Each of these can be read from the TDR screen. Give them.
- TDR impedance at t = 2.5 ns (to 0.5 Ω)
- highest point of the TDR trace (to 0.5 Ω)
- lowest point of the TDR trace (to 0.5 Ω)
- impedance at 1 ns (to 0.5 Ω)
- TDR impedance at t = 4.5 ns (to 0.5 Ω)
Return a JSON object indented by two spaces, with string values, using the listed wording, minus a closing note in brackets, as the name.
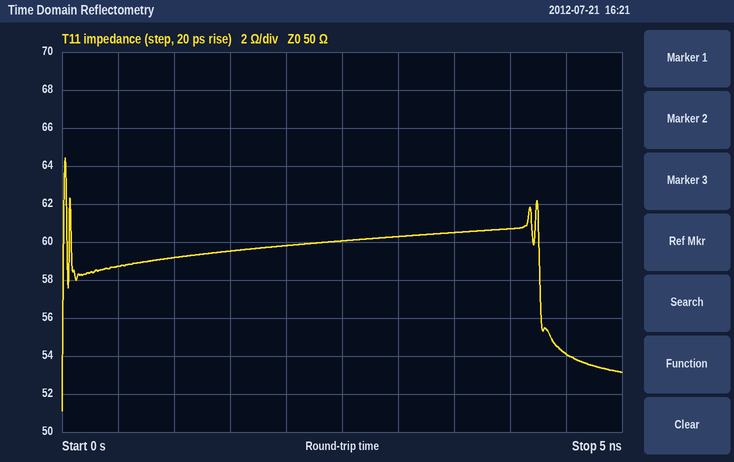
{
  "TDR impedance at t = 2.5 ns": "60.0 Ω",
  "highest point of the TDR trace": "64.5 Ω",
  "lowest point of the TDR trace": "51.0 Ω",
  "impedance at 1 ns": "59.0 Ω",
  "TDR impedance at t = 4.5 ns": "54.0 Ω"
}
